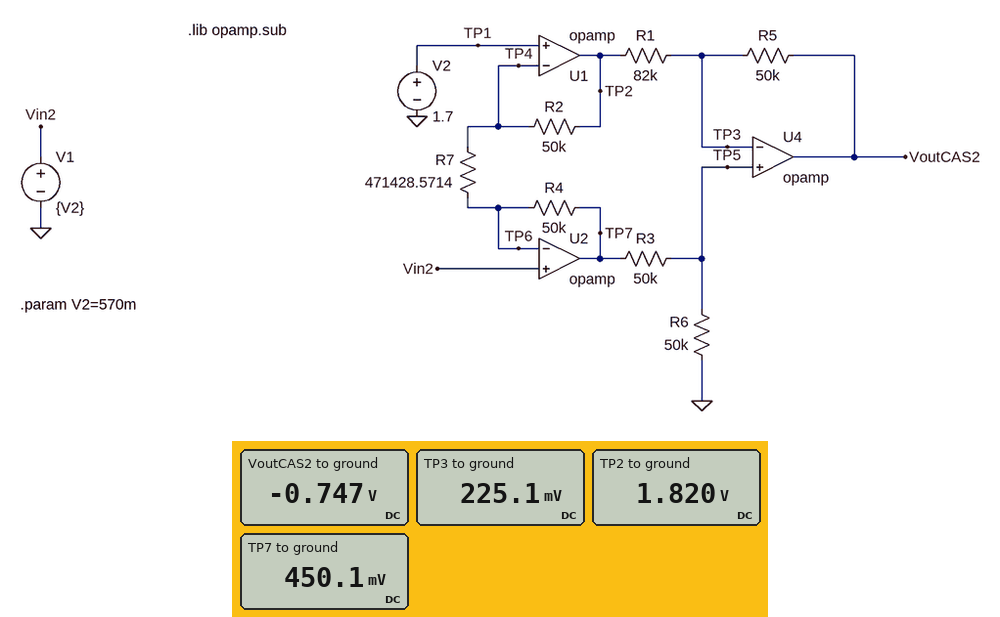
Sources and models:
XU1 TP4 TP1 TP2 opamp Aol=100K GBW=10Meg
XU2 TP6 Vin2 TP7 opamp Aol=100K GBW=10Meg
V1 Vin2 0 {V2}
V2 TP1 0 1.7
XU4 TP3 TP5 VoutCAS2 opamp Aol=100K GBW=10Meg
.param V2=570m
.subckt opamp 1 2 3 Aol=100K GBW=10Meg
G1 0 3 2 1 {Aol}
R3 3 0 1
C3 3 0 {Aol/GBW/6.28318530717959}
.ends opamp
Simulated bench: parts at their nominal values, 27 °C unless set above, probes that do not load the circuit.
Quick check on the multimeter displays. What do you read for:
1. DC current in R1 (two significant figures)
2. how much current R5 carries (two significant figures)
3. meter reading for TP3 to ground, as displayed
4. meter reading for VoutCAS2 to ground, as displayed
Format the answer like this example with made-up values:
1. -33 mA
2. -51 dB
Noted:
1. 19 µA
2. 19 µA
3. 225.1 mV
4. -0.747 V
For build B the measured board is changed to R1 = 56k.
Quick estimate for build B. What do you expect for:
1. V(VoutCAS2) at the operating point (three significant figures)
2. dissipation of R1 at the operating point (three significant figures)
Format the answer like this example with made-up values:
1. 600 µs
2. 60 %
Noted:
1. -1.20 V
2. 45.4 µW
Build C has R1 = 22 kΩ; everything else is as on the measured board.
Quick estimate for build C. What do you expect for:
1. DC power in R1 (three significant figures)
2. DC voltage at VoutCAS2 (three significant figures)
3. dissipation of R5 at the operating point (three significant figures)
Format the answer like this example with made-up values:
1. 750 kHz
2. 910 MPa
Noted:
1. 116 µW
2. -3.40 V
3. 263 µW
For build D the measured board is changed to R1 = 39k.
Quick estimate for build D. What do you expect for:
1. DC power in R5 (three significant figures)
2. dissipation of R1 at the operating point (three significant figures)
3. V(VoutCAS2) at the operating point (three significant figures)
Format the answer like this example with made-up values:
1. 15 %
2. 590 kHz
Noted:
1. 83.6 µW
2. 65.2 µW
3. -1.82 V
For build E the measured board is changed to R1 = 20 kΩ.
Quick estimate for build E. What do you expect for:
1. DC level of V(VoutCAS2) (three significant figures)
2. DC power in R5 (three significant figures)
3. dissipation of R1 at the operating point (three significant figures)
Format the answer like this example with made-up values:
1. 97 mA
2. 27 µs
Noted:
1. -3.76 V
2. 318 µW
3. 127 µW
